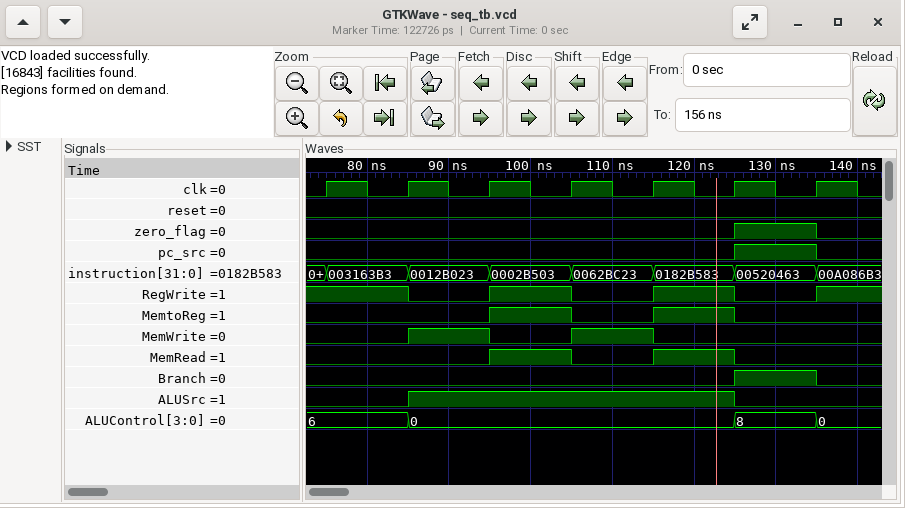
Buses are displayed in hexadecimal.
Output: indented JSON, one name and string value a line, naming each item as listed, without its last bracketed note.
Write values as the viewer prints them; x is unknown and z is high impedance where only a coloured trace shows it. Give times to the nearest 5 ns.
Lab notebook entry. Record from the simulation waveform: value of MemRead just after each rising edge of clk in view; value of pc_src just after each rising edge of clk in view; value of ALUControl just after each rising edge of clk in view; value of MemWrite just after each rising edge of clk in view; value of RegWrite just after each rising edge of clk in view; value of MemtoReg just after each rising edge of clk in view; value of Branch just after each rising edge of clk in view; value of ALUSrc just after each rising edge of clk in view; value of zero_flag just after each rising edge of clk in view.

{
  "value of MemRead just after each rising edge of clk in view": "0 0 1 0 1 0 0",
  "value of pc_src just after each rising edge of clk in view": "0 0 0 0 0 1 0",
  "value of ALUControl just after each rising edge of clk in view": "6, 0, 0, 0, 0, 8, 0",
  "value of MemWrite just after each rising edge of clk in view": "0 1 0 1 0 0 0",
  "value of RegWrite just after each rising edge of clk in view": "1 0 1 0 1 0 1",
  "value of MemtoReg just after each rising edge of clk in view": "0 0 1 0 1 0 0",
  "value of Branch just after each rising edge of clk in view": "0 0 0 0 0 1 0",
  "value of ALUSrc just after each rising edge of clk in view": "0 1 1 1 1 0 0",
  "value of zero_flag just after each rising edge of clk in view": "0 0 0 0 0 1 0"
}
